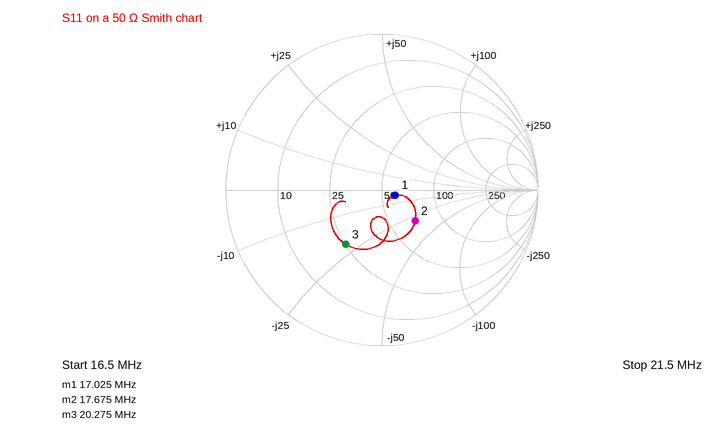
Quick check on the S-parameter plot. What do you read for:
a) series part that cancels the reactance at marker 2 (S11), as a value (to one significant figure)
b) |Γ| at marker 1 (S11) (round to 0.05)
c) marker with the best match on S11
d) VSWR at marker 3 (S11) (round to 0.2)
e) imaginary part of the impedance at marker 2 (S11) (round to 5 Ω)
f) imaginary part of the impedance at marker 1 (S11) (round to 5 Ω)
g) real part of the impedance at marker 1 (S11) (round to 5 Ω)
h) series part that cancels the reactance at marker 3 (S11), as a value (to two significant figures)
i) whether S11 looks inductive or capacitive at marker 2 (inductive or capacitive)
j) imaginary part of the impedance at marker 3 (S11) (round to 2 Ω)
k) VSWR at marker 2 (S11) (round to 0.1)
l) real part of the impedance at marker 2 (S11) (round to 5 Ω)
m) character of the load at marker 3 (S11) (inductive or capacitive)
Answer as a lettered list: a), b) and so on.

a) 300 nH
b) 0.10
c) marker 1
d) 2.4
e) -30 Ω
f) -5 Ω
g) 60 Ω
h) 170 nH
i) capacitive
j) -22 Ω
k) 1.8
l) 70 Ω
m) capacitive
